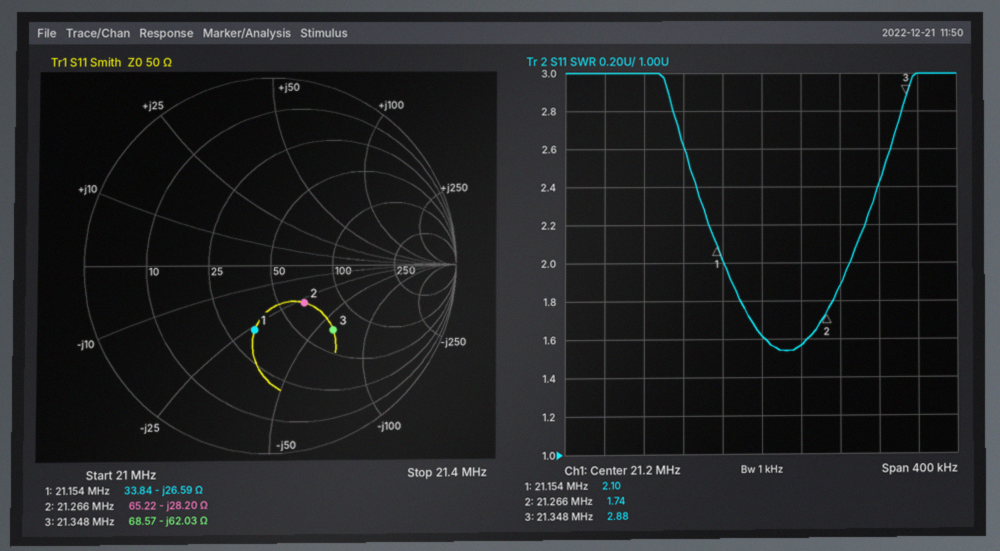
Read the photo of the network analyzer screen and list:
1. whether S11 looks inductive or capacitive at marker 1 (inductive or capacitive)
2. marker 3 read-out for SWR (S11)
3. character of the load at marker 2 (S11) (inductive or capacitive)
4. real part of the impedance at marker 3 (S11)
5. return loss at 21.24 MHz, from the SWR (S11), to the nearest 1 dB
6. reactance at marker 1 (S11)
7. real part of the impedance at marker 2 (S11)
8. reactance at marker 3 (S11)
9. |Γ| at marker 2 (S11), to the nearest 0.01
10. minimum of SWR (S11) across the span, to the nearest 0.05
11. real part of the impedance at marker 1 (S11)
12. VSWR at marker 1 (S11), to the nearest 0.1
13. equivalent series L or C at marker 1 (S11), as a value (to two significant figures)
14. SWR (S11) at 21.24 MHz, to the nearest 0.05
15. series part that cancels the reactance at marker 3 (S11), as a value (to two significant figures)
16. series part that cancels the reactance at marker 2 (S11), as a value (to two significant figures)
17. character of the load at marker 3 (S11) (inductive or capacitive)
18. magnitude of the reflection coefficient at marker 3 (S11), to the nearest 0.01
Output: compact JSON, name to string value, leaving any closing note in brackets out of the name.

{"whether S11 looks inductive or capacitive at marker 1": "capacitive", "marker 3 read-out for SWR": "2.88", "character of the load at marker 2 (S11)": "capacitive", "real part of the impedance at marker 3": "68.57 Ω", "return loss at 21.24 MHz, from the SWR (S11), to the nearest 1 dB": "13 dB", "reactance at marker 1": "-26.59 Ω", "real part of the impedance at marker 2": "65.22 Ω", "reactance at marker 3": "-62.03 Ω", "|Γ| at marker 2 (S11), to the nearest 0.01": "0.27", "minimum of SWR (S11) across the span, to the nearest 0.05": "1.55", "real part of the impedance at marker 1": "33.84 Ω", "VSWR at marker 1 (S11), to the nearest 0.1": "2.1", "equivalent series L or C at marker 1 (S11), as a value": "280 pF", "SWR (S11) at 21.24 MHz, to the nearest 0.05": "1.55", "series part that cancels the reactance at marker 3 (S11), as a value": "460 nH", "series part that cancels the reactance at marker 2 (S11), as a value": "210 nH", "character of the load at marker 3 (S11)": "capacitive", "magnitude of the reflection coefficient at marker 3 (S11), to the nearest 0.01": "0.48"}
